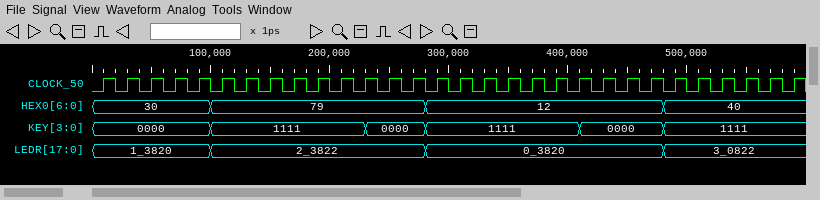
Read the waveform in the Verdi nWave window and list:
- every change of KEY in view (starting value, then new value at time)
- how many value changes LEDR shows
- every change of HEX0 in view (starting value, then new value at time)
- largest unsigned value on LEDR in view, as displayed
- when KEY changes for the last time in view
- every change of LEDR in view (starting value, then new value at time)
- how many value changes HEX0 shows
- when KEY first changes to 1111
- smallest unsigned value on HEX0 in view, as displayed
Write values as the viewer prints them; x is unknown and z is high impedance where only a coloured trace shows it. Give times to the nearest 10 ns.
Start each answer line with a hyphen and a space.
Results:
- 0000, 1111 at 100 ns, 0000 at 230 ns, 1111 at 280 ns, 0000 at 410 ns, 1111 at 480 ns
- 3
- 30, 79 at 100 ns, 12 at 280 ns, 40 at 480 ns
- 3_0822
- 480 ns
- 1_3820, 2_3822 at 100 ns, 0_3820 at 280 ns, 3_0822 at 480 ns
- 3
- 100 ns
- 12
